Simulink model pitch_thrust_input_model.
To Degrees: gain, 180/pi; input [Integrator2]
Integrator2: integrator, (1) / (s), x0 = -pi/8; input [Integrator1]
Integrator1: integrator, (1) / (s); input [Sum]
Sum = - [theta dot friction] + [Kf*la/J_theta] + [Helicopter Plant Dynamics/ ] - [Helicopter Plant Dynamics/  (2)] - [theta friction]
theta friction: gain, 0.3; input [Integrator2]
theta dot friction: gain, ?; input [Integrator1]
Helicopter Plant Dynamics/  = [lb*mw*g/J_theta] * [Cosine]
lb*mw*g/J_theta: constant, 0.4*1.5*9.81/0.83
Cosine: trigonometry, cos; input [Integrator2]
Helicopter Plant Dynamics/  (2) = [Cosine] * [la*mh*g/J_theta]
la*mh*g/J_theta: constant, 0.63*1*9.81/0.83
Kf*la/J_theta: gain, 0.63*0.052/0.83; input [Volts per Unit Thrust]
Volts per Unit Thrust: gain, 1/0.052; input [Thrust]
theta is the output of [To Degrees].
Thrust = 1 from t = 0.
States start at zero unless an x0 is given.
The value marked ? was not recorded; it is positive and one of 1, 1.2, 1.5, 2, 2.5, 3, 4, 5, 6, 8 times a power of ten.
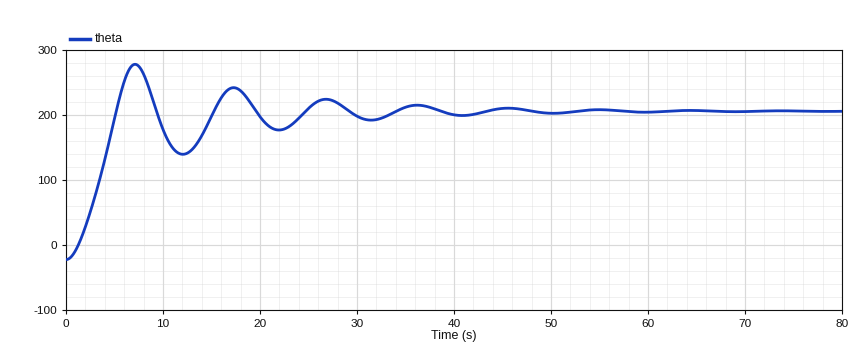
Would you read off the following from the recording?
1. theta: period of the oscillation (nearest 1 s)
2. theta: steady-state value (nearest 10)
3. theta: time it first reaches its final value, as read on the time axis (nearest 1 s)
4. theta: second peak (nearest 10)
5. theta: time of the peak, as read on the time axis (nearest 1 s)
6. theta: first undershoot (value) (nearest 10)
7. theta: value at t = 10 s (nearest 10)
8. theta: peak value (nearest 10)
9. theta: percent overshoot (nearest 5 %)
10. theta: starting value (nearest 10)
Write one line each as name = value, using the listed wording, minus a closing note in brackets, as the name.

theta: period of the oscillation = 10 s
theta: steady-state value = 210
theta: time it first reaches its final value, as read on the time axis = 5 s
theta: second peak = 240
theta: time of the peak, as read on the time axis = 7 s
theta: first undershoot (value) = 140
theta: value at t = 10 s = 180
theta: peak value = 280
theta: percent overshoot = 30 %
theta: starting value = -20
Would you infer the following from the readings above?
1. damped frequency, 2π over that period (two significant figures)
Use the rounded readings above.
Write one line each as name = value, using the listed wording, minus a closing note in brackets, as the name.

damped frequency, 2π over that period = 0.63 rad/s
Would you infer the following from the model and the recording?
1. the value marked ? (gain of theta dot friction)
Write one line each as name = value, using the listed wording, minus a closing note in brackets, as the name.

the value marked ? = 0.15
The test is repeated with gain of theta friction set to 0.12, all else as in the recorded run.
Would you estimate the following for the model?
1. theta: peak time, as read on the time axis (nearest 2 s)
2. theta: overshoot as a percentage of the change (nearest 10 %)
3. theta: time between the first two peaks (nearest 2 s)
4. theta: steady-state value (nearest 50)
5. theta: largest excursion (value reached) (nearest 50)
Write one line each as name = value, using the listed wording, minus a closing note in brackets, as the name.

theta: peak time, as read on the time axis = 12 s
theta: overshoot as a percentage of the change = 90 %
theta: time between the first two peaks = 20 s
theta: steady-state value = 300
theta: largest excursion (value reached) = 600
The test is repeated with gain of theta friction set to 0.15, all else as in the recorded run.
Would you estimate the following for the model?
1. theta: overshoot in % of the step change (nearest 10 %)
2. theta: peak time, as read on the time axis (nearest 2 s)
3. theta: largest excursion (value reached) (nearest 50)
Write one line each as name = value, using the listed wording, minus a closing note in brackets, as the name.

theta: overshoot in % of the step change = 50 %
theta: peak time, as read on the time axis = 8 s
theta: largest excursion (value reached) = 400
